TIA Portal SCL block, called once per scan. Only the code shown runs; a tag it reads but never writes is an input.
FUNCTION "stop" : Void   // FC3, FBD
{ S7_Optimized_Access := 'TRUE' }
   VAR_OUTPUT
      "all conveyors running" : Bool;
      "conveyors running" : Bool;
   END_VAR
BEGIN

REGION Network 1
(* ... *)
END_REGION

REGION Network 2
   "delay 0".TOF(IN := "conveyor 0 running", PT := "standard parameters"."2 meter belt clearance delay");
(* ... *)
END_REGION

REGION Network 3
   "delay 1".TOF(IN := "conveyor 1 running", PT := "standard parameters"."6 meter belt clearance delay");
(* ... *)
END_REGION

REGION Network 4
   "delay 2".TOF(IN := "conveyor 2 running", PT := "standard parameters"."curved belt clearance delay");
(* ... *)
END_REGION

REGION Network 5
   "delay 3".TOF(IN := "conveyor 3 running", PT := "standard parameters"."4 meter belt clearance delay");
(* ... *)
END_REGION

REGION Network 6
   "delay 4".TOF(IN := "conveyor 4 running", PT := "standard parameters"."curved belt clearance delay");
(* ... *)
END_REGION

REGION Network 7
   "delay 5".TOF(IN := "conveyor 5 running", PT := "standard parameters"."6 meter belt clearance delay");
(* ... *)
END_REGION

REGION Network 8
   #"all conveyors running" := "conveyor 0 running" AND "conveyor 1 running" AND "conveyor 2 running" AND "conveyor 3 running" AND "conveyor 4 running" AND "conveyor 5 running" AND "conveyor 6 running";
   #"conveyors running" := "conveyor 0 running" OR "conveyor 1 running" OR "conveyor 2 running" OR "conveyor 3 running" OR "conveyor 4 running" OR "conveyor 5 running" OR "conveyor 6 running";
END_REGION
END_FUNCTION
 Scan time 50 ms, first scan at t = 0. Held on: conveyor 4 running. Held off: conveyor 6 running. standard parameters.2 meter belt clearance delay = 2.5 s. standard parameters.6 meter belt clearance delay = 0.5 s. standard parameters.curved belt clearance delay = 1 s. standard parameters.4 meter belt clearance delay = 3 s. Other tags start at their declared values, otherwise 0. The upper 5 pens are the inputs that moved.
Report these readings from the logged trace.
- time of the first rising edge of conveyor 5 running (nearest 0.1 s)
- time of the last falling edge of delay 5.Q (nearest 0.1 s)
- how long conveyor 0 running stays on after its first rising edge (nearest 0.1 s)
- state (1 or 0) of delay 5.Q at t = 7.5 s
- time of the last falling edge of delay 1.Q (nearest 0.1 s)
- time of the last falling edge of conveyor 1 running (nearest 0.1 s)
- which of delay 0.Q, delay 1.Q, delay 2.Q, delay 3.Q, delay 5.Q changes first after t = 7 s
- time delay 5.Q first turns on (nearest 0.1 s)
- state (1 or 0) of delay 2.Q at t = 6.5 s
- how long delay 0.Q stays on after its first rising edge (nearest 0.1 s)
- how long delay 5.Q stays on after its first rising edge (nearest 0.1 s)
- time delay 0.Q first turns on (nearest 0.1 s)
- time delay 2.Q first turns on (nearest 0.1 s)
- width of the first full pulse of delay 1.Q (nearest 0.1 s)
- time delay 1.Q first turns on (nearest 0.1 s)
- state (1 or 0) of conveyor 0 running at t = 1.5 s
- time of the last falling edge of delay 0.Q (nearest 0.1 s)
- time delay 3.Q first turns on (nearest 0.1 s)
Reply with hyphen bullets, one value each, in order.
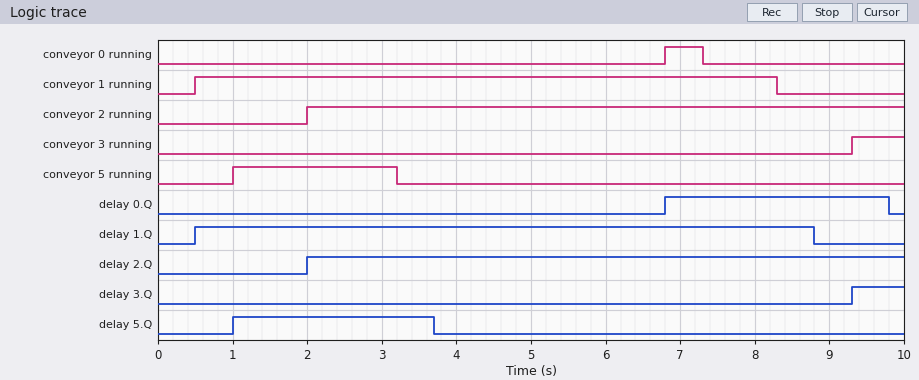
- 1.0 s
- 3.7 s
- 0.5 s
- 0
- 8.8 s
- 8.3 s
- delay 1.Q
- 1.0 s
- 1
- 3.0 s
- 2.7 s
- 6.8 s
- 2.0 s
- 8.3 s
- 0.5 s
- 0
- 9.8 s
- 9.3 s
